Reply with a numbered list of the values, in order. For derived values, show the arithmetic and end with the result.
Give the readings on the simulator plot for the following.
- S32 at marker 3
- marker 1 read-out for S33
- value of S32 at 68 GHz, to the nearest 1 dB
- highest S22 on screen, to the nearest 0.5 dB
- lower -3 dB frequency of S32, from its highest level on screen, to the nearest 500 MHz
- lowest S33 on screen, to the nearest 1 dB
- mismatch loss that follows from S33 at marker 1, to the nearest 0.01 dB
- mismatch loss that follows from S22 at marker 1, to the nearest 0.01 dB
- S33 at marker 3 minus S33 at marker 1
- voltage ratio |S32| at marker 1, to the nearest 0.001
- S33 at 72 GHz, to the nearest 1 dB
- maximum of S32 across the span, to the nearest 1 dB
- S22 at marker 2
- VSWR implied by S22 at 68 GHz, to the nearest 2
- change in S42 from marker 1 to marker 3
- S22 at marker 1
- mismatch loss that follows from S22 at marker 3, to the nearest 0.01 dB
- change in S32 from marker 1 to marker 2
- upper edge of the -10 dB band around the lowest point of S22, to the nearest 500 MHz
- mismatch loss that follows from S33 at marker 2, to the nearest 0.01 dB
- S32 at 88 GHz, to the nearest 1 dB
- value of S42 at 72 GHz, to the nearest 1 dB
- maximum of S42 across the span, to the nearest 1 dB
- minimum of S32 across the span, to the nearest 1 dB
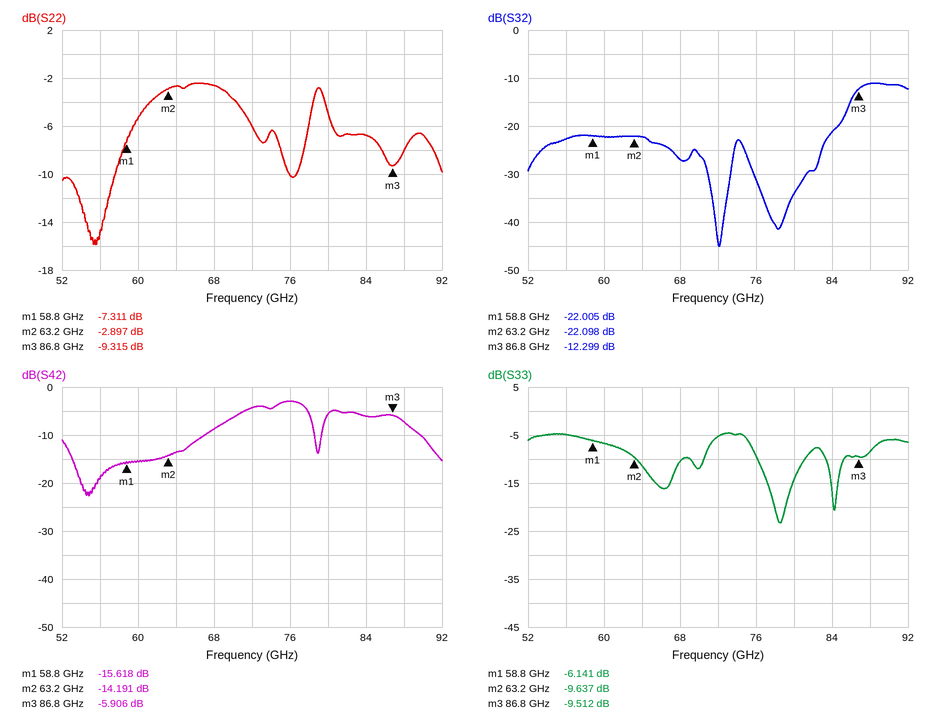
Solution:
1. -12.299 dB
2. -6.141 dB
3. -27 dB
4. -2.5 dB
5. 86.0 GHz
6. -23 dB
7. −10 log10(1 − 10^(-6.141/10)) ≈ 1.21 dB
8. −10 log10(1 − 10^(-7.311/10)) ≈ 0.89 dB
9. -9.512 − (-6.141) = -3.371 dB
10. 10^(-22.005/20) ≈ 0.079
11. -5 dB
12. -11 dB
13. -2.897 dB
14. |Γ| = 10^(-2.5/20) = 0.7499; VSWR = (1 + 0.7499)/(1 − 0.7499) ≈ 7.00, so 6 to the nearest 2
15. -5.906 − (-15.618) = 9.712 dB
16. -7.311 dB
17. −10 log10(1 − 10^(-9.315/10)) ≈ 0.54 dB
18. -22.098 − (-22.005) = -0.093 dB
19. 57.5 GHz
20. −10 log10(1 − 10^(-9.637/10)) ≈ 0.50 dB
21. -11 dB
22. -4 dB
23. -3 dB
24. -45 dB
